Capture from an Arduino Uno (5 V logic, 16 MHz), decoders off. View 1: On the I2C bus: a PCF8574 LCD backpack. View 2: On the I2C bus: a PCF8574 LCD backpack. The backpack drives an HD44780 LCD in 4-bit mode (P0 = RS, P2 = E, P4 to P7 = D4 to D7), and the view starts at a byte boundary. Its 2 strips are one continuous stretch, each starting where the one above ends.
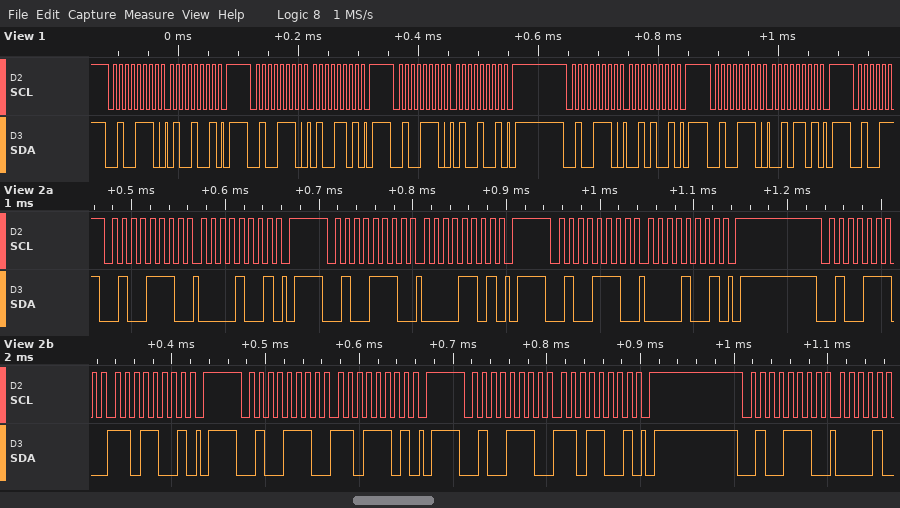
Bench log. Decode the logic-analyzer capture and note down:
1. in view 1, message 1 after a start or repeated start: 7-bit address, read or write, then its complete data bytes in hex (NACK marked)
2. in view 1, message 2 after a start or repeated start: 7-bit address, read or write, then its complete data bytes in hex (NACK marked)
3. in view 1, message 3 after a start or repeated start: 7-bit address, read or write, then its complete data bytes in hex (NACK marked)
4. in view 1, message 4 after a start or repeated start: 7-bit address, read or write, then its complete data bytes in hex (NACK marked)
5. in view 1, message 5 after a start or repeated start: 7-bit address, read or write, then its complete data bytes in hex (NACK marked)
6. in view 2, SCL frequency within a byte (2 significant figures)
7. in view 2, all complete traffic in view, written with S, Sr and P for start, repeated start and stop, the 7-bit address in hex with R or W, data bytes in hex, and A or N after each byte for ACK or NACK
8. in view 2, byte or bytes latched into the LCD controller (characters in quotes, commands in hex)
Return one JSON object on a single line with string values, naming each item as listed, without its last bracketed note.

{"in view 1, message 1 after a start or repeated start: 7-bit address, read or write, then its complete data bytes in hex": "0x27 write: 49", "in view 1, message 2 after a start or repeated start: 7-bit address, read or write, then its complete data bytes in hex": "0x27 write: 4D", "in view 1, message 3 after a start or repeated start: 7-bit address, read or write, then its complete data bytes in hex": "0x27 write: 49", "in view 1, message 4 after a start or repeated start: 7-bit address, read or write, then its complete data bytes in hex": "0x27 write: 29", "in view 1, message 5 after a start or repeated start: 7-bit address, read or write, then its complete data bytes in hex": "0x27 write: 2D", "in view 2, SCL frequency within a byte": "100 kHz", "in view 2, all complete traffic in view, written with S, Sr and P for start, repeated start and stop, the 7-bit address in hex with R or W, data bytes in hex, and A or N after each byte for ACK or NACK": "S 27W A 09 A P S 27W A 0D A P S 27W A 09 A P S 27W A D9 A P S 27W A DD A P S 27W A D9 A P S 27W A", "in view 2, byte or bytes latched into the LCD controller": "data 0x0D"}
